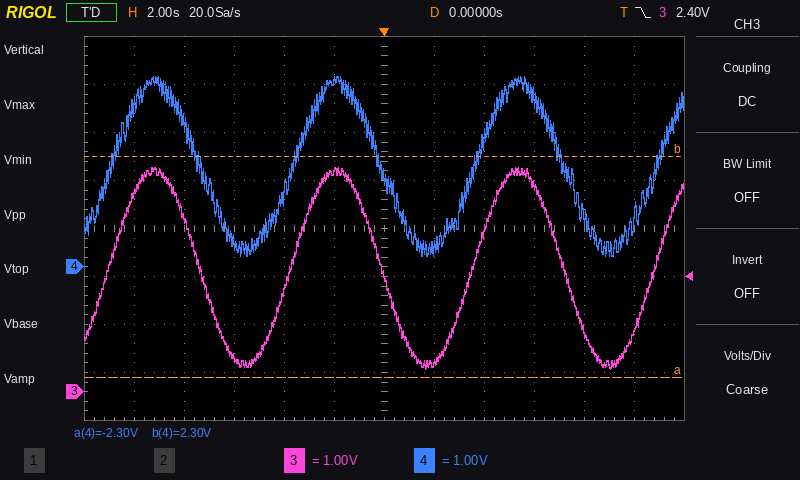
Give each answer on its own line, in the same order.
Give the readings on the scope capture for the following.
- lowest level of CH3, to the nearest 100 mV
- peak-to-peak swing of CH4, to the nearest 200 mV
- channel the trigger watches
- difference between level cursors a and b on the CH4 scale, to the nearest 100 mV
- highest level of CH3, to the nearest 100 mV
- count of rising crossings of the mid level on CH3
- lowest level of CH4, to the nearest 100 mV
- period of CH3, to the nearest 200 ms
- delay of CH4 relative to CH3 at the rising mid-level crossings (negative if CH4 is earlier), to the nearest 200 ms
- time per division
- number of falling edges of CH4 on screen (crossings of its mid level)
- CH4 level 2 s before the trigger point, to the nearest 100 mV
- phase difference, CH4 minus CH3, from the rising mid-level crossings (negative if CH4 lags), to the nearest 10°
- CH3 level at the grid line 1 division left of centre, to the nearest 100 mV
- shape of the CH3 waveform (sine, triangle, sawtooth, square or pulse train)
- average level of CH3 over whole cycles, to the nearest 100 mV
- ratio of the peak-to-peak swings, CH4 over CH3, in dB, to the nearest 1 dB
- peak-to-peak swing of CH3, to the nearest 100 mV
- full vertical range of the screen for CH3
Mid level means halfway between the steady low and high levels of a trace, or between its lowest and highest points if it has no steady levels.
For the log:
500 mV
3.8 V
CH3
4.6 V
4.7 V
4
200 mV
7.2 s
0.0 s
2 s
3
3.9 V
0°
4.6 V
sine
2.6 V
-1 dB
4.2 V
8 V
